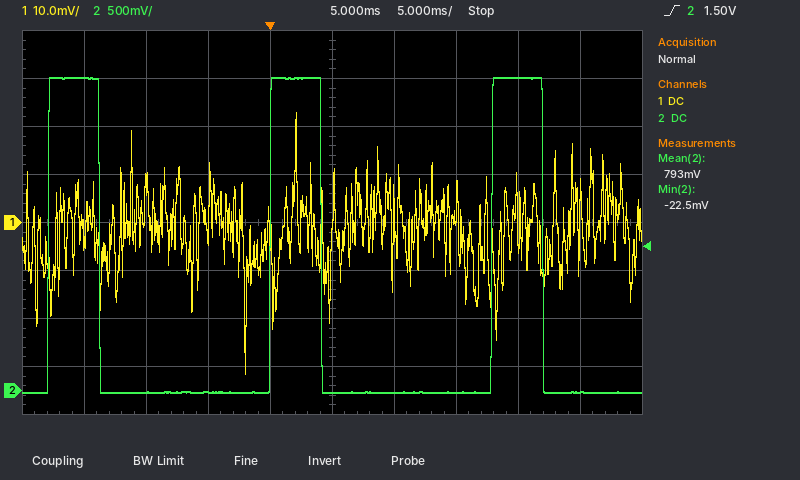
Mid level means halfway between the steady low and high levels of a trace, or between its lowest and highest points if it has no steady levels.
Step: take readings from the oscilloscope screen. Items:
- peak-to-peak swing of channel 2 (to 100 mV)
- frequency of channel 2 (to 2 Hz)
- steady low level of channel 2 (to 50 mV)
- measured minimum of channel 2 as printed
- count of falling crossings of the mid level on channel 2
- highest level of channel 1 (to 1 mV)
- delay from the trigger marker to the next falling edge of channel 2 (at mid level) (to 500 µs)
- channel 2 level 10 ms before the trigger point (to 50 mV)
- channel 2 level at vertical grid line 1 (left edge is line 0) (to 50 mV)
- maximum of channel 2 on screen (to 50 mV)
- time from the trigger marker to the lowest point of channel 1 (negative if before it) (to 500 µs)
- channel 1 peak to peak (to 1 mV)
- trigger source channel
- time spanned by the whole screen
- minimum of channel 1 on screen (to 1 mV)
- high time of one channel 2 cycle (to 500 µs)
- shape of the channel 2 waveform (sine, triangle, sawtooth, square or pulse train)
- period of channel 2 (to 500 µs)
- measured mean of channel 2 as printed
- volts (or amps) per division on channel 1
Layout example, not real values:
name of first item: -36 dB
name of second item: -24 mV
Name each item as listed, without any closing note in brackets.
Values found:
peak-to-peak swing of channel 2: 3.30 V
frequency of channel 2: 56 Hz
steady low level of channel 2: 0 mV
measured minimum of channel 2 as printed: -22.5 mV
count of falling crossings of the mid level on channel 2: 3
highest level of channel 1: 23 mV
delay from the trigger marker to the next falling edge of channel 2 (at mid level): 4.0 ms
channel 2 level 10 ms before the trigger point: 0 mV
channel 2 level at vertical grid line 1 (left edge is line 0): 3.25 V
maximum of channel 2 on screen: 3.25 V
time from the trigger marker to the lowest point of channel 1 (negative if before it): -2.0 ms
channel 1 peak to peak: 54 mV
trigger source channel: channel 2
time spanned by the whole screen: 50 ms
minimum of channel 1 on screen: -31 mV
high time of one channel 2 cycle: 4.0 ms
shape of the channel 2 waveform: pulse train
period of channel 2: 18.0 ms
measured mean of channel 2 as printed: 793 mV
volts (or amps) per division on channel 1: 10 mV
